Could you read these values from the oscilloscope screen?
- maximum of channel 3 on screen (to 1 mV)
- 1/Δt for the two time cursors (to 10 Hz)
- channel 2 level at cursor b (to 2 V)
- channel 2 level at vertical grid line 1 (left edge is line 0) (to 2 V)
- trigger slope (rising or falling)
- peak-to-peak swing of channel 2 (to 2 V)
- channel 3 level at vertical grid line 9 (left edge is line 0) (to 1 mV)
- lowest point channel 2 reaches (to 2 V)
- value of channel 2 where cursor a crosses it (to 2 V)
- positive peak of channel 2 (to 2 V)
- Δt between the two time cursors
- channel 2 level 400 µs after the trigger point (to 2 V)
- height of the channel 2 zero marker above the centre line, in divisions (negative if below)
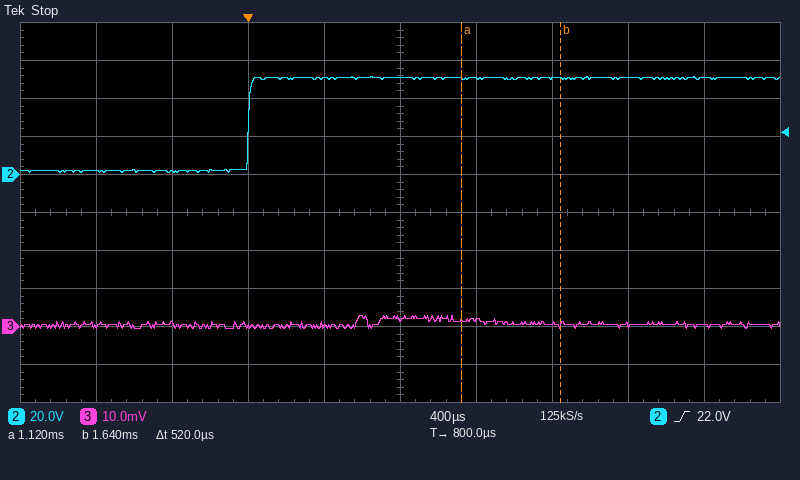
3 mV
1.92 kHz
50 V
2 V
rising
50 V
0 mV
2 V
50 V
52 V
520 µs
50 V
+1.0 div
